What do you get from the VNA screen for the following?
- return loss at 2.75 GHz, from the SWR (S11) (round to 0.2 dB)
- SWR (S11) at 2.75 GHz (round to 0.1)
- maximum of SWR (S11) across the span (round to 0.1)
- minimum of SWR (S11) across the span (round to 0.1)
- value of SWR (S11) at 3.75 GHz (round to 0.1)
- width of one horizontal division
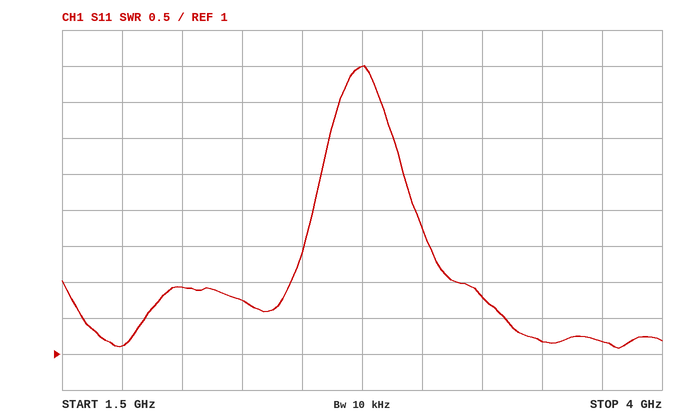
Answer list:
3.6 dB
5.0
5.0
1.1
1.2
250 MHz
